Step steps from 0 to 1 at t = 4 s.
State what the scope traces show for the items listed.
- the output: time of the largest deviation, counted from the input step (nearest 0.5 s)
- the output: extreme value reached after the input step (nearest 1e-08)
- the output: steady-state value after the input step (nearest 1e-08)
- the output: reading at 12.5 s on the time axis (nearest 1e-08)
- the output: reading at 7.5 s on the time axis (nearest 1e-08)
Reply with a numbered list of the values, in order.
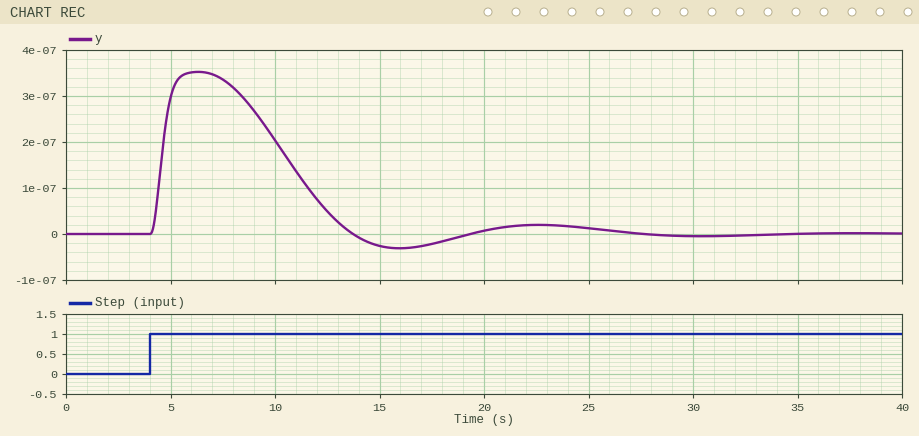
1. 2.5 s
2. 0.00000035
3. 0.00000000
4. 0.00000005
5. 0.00000034
